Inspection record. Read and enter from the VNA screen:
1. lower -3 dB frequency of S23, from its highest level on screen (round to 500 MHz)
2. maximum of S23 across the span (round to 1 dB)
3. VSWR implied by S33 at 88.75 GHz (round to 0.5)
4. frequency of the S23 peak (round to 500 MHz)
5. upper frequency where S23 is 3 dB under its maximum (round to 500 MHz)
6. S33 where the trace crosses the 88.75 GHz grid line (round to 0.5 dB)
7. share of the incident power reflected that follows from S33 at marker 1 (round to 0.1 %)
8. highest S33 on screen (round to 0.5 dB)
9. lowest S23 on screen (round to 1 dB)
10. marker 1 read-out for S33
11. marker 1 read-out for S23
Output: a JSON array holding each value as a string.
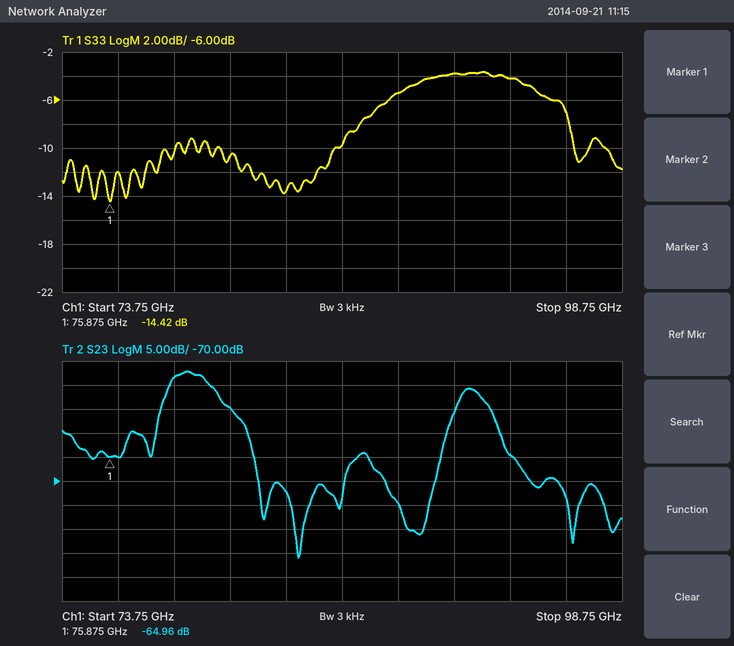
["78.5 GHz", "-47 dB", "3.5", "79.5 GHz", "80.5 GHz", "-5.5 dB", "3.6 %", "-3.5 dB", "-86 dB", "-14.42 dB", "-64.96 dB"]
